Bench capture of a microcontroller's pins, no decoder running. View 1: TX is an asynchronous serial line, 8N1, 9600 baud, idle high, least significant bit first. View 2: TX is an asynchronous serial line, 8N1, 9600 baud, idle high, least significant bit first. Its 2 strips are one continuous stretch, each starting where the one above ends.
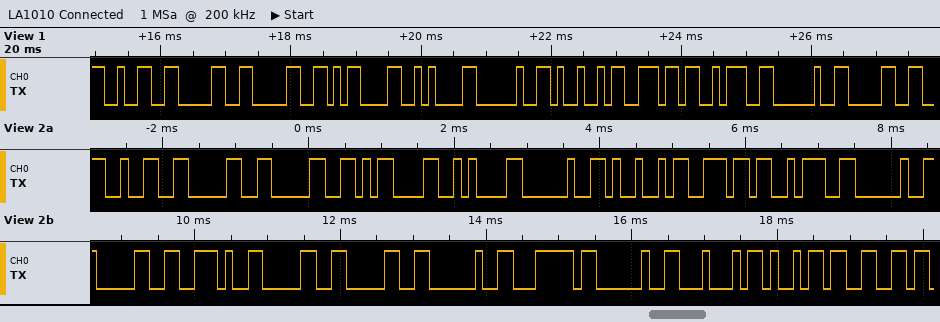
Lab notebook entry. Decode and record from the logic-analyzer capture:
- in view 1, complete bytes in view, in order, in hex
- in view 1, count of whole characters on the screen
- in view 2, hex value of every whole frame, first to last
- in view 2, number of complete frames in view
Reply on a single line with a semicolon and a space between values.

32 30 30 0D 0A 20 49 6E 3A 20 30; 11; 32 30 30 0D 0A 20 49 6E 3A 20 30 2E 30 30 20 7C 20 44 69 66; 20
